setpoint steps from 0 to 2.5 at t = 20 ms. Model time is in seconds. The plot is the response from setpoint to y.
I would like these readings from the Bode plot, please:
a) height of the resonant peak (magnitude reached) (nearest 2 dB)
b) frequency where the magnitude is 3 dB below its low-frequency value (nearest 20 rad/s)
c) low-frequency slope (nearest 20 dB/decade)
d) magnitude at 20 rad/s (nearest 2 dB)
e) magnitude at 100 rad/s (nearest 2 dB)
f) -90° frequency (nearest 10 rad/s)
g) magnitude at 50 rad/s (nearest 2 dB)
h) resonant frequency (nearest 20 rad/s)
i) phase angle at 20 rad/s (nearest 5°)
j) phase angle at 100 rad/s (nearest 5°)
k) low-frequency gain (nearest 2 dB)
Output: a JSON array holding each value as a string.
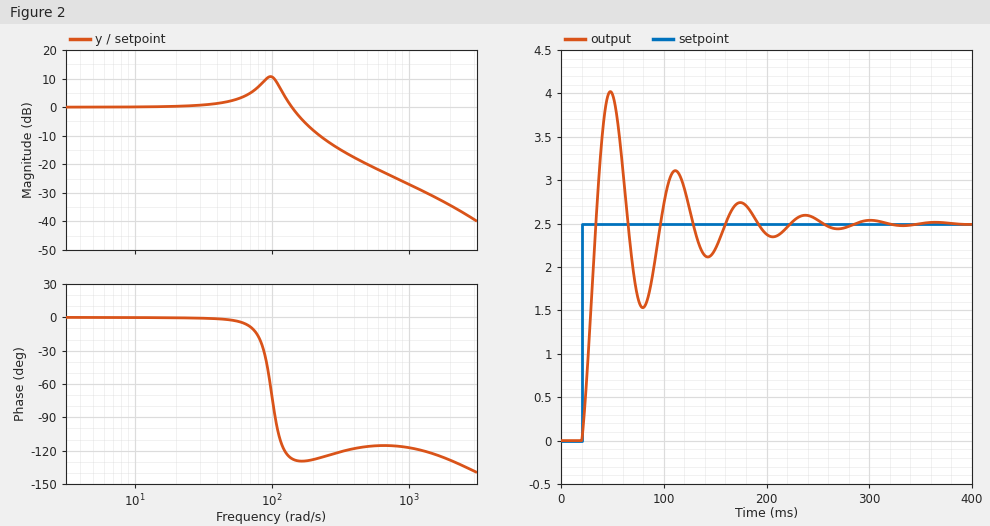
["10 dB", "160 rad/s", "0 dB/decade", "0 dB", "10 dB", "110 rad/s", "2 dB", "100 rad/s", "0°", "-70°", "0 dB"]
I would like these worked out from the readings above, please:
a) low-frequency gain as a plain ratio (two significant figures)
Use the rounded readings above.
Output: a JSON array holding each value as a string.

["1.0"]
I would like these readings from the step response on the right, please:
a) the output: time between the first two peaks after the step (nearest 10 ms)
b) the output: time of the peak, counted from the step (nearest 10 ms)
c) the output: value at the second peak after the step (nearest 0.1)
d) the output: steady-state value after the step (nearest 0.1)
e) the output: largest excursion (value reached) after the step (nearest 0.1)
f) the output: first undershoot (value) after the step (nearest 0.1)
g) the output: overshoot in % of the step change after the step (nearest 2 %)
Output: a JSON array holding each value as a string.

["60 ms", "30 ms", "3.1", "2.5", "4.0", "1.5", "60 %"]
